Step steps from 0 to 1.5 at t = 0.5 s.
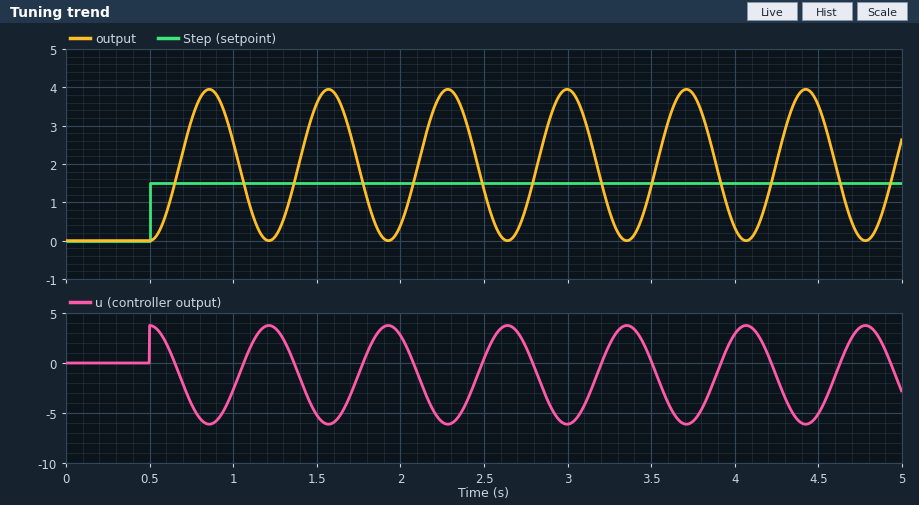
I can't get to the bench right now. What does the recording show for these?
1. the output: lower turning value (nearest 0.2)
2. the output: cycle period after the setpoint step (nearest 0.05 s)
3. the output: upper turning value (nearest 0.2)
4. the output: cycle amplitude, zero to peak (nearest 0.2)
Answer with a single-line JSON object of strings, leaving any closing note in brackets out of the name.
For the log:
{"the output: lower turning value": "0.0", "the output: cycle period after the setpoint step": "0.70 s", "the output: upper turning value": "4.0", "the output: cycle amplitude, zero to peak": "2.0"}
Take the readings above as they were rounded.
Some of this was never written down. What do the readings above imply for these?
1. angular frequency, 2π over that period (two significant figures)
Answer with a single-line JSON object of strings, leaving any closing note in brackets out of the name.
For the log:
{"angular frequency, 2π over that period": "9.0 rad/s"}
